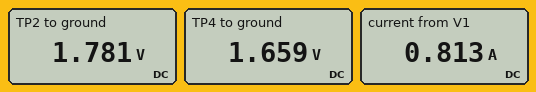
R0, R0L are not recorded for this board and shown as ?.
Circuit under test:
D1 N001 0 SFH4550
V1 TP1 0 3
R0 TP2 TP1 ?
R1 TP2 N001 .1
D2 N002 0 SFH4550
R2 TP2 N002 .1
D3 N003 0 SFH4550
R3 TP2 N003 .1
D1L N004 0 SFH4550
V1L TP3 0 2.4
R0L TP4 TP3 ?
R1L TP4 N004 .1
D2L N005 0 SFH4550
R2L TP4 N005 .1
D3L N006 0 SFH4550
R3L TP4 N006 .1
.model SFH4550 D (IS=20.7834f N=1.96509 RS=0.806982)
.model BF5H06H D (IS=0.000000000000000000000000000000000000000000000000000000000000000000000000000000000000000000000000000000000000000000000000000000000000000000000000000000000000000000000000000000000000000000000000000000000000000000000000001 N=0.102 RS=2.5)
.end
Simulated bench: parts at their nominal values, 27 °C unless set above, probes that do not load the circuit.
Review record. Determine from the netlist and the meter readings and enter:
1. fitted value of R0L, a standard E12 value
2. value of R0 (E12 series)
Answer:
1.5 Ω
1.5 Ω
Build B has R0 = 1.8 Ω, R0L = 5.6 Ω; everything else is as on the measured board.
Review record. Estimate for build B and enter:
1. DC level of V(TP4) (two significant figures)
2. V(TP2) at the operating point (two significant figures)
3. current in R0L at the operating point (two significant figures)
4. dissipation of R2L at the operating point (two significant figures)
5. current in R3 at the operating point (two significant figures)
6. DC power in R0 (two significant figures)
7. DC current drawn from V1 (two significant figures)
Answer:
1.5 V
1.7 V
160 mA
290 µW
230 mA
880 mW
700 mA
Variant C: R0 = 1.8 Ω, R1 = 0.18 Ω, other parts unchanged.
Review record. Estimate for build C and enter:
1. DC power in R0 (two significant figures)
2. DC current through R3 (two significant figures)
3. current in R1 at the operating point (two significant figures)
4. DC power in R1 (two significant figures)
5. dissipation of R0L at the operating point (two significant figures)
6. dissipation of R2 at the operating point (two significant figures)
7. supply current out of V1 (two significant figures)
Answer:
880 mW
240 mA
220 mA
8.9 mW
370 mW
5.7 mW
700 mA
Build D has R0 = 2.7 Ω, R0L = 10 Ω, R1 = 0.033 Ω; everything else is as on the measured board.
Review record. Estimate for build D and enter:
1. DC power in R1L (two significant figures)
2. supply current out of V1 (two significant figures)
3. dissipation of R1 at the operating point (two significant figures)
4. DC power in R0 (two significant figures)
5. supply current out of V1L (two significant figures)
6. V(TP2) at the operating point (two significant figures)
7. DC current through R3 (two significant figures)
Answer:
99 µW
500 mA
980 µW
670 mW
95 mA
1.7 V
160 mA
